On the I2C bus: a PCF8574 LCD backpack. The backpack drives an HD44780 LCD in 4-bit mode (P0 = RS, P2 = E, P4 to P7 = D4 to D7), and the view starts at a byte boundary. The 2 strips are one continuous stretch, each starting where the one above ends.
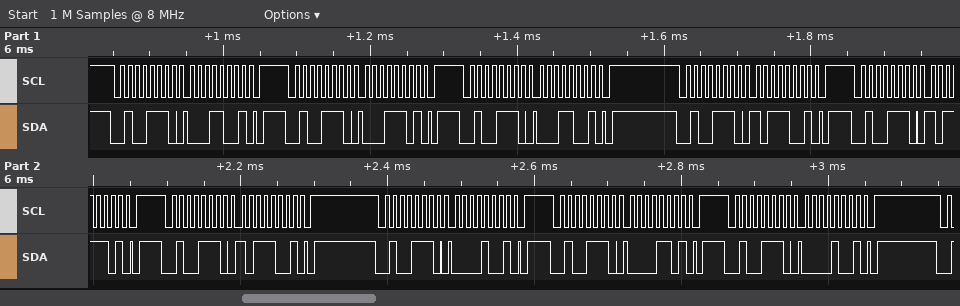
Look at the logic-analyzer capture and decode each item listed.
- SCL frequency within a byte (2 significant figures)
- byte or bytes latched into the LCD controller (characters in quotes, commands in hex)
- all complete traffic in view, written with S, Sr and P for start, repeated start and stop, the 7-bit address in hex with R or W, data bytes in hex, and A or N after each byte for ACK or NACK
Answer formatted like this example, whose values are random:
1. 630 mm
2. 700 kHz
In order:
1. 100 kHz
2. data 0x1B
3. S 27W A 19 A P S 27W A 1D A P S 27W A 19 A P S 27W A B9 A P S 27W A BD A P S 27W A B9 A P S 27W A 09 A P S 27W A 0D A P S 27W A 09 A P
